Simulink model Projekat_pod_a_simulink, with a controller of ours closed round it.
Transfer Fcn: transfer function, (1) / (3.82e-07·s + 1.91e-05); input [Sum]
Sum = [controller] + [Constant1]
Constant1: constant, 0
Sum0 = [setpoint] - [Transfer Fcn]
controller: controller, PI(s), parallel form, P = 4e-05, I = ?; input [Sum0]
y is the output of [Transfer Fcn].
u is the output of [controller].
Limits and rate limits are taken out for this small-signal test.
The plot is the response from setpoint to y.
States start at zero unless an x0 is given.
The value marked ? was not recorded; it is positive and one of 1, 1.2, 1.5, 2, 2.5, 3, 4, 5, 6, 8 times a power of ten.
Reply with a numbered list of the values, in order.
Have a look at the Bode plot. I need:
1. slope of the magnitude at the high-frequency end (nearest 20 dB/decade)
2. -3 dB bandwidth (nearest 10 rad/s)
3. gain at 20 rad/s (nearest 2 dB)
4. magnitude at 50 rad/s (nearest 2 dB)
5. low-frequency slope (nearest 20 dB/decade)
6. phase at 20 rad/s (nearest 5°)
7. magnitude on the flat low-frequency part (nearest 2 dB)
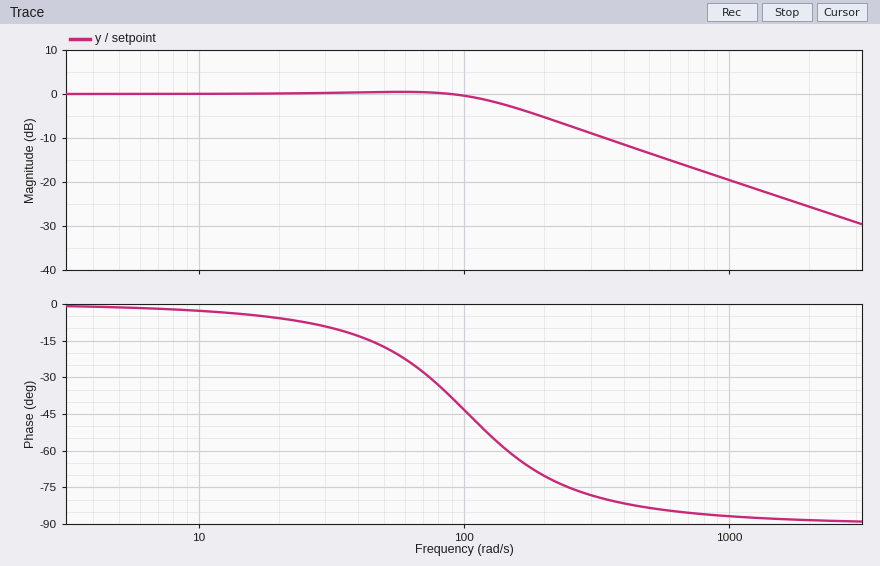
1. -20 dB/decade
2. 150 rad/s
3. 0 dB
4. 0 dB
5. 0 dB/decade
6. -5°
7. 0 dB
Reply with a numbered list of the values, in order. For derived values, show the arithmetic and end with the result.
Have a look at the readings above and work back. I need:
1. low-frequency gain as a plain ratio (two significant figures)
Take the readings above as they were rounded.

1. 10^(0 / 20) = 1.0
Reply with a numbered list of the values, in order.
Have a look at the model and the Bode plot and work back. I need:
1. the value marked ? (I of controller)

1. 0.004
